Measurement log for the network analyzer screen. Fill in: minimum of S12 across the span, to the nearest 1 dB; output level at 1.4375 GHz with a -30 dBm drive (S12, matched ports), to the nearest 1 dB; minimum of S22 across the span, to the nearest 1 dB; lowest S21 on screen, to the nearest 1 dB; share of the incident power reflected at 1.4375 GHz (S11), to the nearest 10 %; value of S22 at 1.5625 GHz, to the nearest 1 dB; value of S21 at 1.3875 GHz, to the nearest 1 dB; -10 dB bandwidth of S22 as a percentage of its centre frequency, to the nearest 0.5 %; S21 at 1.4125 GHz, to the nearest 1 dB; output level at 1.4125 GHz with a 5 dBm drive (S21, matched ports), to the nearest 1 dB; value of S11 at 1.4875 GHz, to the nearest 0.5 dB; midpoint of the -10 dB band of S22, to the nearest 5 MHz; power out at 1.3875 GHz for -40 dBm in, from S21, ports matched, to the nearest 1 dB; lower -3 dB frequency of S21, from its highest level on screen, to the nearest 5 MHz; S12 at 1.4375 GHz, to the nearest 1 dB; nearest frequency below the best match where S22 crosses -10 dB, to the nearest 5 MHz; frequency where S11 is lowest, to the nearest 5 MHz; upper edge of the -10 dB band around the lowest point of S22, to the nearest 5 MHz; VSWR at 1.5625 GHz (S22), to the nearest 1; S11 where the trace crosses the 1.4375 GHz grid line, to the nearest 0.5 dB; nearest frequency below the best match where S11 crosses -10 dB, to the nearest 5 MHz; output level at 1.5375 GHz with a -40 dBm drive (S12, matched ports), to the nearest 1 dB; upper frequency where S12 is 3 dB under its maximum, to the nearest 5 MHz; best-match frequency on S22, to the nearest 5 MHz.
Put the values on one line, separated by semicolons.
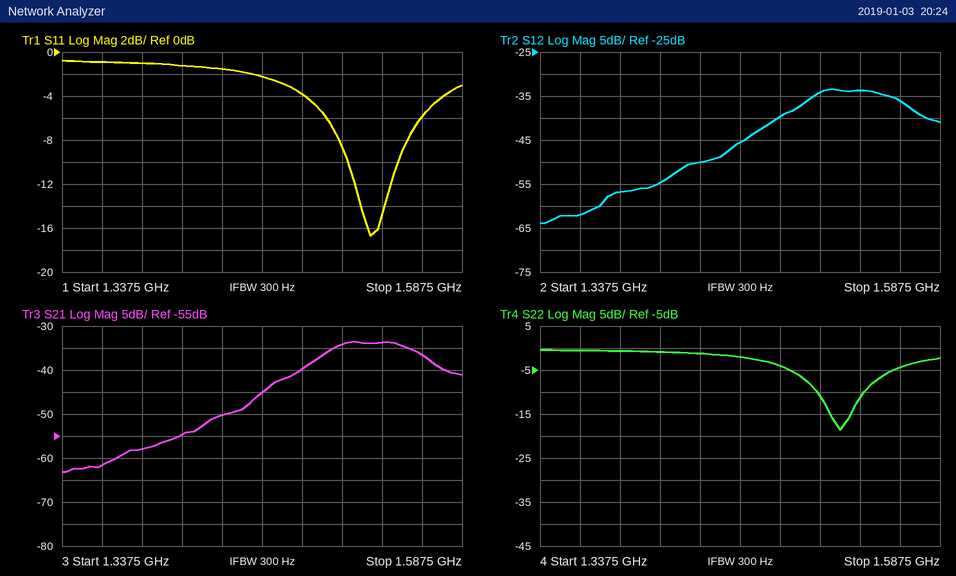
-64 dB; -80 dBm; -19 dB; -63 dB; 70 %; -4 dB; -58 dB; 2.0 %; -55 dB; -50 dBm; -4.0 dB; 1.525 GHz; -98 dBm; 1.500 GHz; -50 dB; 1.510 GHz; 1.530 GHz; 1.540 GHz; 4; -1.5 dB; 1.515 GHz; -74 dBm; 1.565 GHz; 1.525 GHz
